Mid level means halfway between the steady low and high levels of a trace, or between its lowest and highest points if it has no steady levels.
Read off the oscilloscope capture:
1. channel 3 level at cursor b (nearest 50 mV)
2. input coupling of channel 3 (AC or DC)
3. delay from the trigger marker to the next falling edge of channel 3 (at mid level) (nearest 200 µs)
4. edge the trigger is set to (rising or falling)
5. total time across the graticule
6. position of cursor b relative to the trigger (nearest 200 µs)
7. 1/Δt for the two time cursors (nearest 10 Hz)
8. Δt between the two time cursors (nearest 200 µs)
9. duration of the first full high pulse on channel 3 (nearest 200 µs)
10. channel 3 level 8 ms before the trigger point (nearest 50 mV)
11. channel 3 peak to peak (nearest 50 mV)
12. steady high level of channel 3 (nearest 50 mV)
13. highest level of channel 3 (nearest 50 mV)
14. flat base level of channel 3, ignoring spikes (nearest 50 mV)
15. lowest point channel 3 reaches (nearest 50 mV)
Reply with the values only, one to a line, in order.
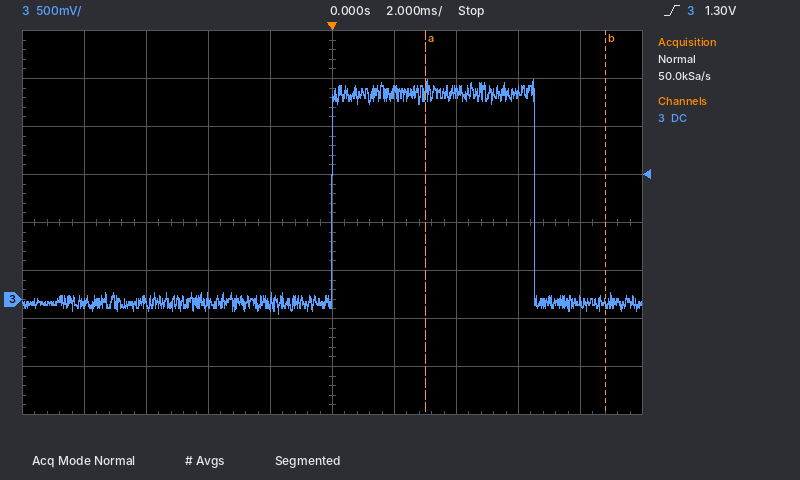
-50 mV
DC
6.6 ms
rising
20 ms
+8.8 ms
170 Hz
5.8 ms
6.6 ms
-50 mV
2.45 V
2.15 V
2.30 V
-50 mV
-150 mV
